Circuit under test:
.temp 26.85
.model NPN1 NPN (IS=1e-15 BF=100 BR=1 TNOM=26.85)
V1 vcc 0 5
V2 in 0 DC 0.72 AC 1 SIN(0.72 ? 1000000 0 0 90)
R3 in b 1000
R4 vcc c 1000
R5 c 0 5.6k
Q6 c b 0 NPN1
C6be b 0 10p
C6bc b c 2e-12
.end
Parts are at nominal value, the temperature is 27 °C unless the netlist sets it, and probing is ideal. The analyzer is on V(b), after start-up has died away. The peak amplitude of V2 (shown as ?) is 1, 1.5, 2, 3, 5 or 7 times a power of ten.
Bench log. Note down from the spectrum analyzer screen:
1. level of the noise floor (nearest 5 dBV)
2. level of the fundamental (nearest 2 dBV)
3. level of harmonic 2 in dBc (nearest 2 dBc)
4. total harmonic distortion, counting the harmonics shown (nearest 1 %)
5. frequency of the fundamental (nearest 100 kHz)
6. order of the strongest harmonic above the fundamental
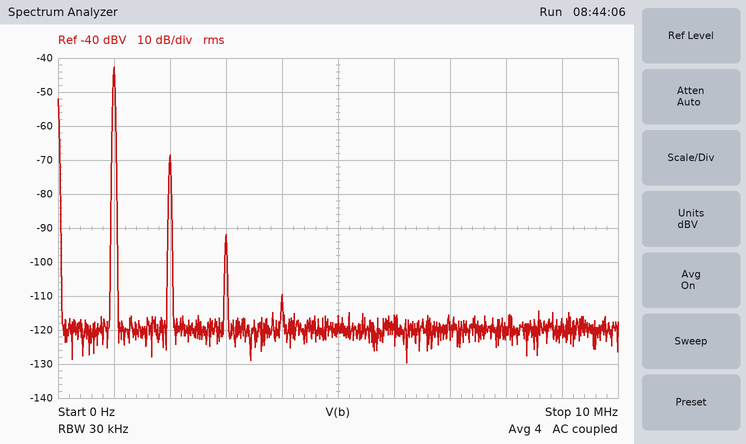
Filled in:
-120 dBV
-42 dBV
-26 dBc
5 %
1.0 MHz
2
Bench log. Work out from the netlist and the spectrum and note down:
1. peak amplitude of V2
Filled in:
15 mV
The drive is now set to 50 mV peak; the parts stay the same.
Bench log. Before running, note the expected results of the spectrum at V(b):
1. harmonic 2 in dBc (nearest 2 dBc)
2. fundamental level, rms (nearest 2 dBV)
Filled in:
-16 dBc
-32 dBV
